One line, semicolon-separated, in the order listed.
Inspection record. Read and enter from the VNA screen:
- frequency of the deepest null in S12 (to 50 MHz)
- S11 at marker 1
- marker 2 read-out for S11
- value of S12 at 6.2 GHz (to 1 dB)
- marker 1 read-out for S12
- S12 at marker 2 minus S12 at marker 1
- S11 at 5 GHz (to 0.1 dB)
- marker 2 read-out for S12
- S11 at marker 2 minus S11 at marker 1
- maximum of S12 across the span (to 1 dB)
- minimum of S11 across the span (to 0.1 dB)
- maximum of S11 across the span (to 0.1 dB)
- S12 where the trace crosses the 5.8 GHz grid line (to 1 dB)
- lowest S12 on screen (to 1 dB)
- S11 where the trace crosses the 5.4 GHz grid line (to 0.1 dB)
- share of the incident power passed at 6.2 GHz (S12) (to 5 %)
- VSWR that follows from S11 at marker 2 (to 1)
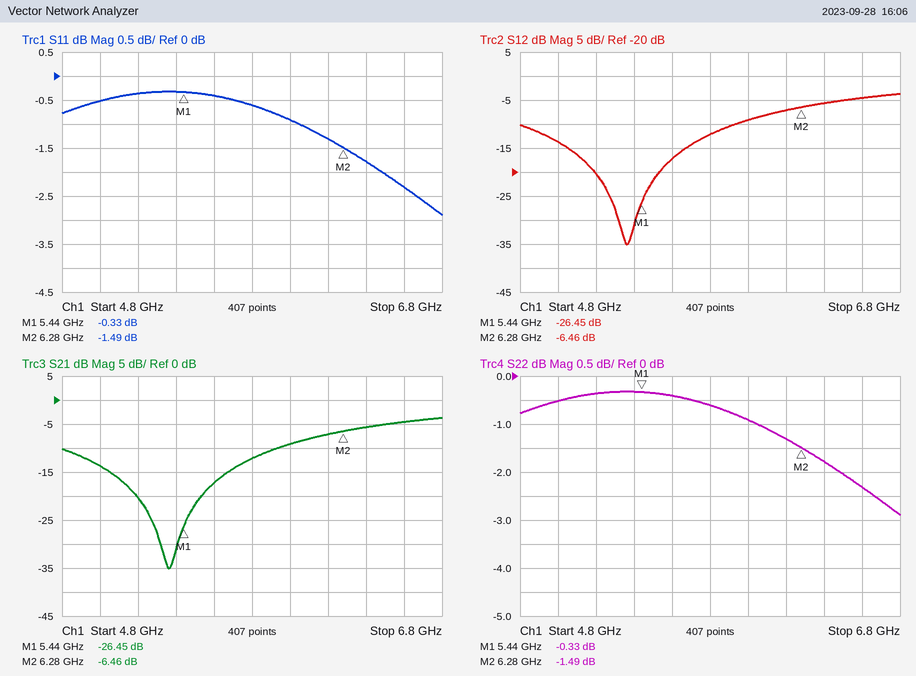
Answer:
5.35 GHz; -0.33 dB; -1.49 dB; -7 dB; -26.45 dB; 19.99 dB; -0.5 dB; -6.46 dB; -1.16 dB; -4 dB; -2.9 dB; -0.3 dB; -12 dB; -35 dB; -0.3 dB; 20 %; 12
